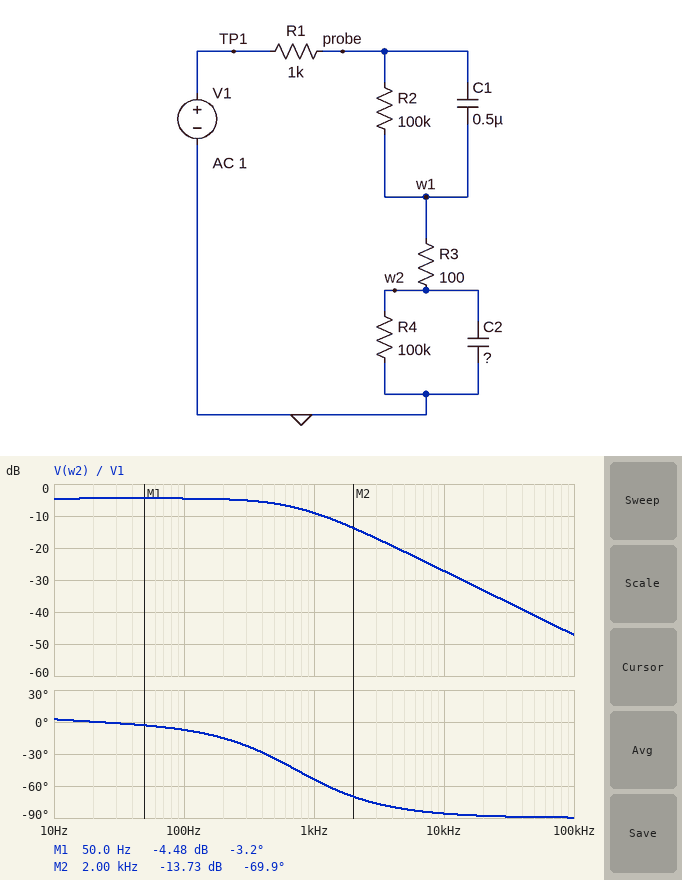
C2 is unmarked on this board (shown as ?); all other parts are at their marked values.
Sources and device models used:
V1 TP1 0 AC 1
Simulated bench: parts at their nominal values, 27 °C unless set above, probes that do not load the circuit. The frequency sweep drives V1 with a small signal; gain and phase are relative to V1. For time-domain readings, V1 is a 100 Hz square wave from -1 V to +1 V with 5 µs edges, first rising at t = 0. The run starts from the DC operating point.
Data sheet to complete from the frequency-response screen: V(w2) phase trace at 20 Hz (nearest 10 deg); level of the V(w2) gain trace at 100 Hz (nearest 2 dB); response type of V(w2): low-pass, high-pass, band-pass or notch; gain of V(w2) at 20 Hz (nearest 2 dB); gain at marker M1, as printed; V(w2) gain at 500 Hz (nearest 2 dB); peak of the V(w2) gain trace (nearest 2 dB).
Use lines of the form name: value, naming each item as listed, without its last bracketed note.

V(w2) phase trace at 20 Hz: 0 deg
level of the V(w2) gain trace at 100 Hz: -4 dB
response type of V(w2): low-pass, high-pass, band-pass or notch: low-pass
gain of V(w2) at 20 Hz: -4 dB
gain at marker M1, as printed: -4.48 dB
V(w2) gain at 500 Hz: -6 dB
peak of the V(w2) gain trace: -4 dB
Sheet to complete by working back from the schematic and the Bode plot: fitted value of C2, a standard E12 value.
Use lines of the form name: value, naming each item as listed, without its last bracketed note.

fitted value of C2, a standard E12 value: 330 nF
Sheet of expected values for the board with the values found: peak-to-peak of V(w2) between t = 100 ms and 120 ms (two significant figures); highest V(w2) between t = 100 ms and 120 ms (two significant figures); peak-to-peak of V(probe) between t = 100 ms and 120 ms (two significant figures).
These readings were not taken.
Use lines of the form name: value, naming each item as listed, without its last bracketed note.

peak-to-peak of V(w2) between t = 100 ms and 120 ms: 1.2 V
highest V(w2) between t = 100 ms and 120 ms: 610 mV
peak-to-peak of V(probe) between t = 100 ms and 120 ms: 2.0 V
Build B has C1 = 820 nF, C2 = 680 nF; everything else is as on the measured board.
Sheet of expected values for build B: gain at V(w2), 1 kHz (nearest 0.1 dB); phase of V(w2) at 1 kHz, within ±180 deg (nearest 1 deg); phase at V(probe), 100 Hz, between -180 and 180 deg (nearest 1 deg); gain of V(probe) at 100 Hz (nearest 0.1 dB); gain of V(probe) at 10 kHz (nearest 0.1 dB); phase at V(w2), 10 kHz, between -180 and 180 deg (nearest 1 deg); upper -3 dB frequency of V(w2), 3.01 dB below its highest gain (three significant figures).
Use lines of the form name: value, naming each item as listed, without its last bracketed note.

gain at V(w2), 1 kHz: -14.1 dB
phase of V(w2) at 1 kHz, within ±180 deg: -69 deg
phase at V(probe), 100 Hz, between -180 and 180 deg: -13 deg
gain of V(probe) at 100 Hz: -0.3 dB
gain of V(probe) at 10 kHz: -20.1 dB
phase at V(w2), 10 kHz, between -180 and 180 deg: -88 deg
upper -3 dB frequency of V(w2), 3.01 dB below its highest gain: 393 Hz
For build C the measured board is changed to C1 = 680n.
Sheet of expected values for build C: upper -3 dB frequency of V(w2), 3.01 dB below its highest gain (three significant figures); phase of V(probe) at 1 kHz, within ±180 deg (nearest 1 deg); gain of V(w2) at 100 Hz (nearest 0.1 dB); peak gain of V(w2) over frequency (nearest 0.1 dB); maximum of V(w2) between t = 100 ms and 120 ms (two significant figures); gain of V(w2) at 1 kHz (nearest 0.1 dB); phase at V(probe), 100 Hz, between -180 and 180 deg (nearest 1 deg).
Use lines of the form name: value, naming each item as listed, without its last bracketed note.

upper -3 dB frequency of V(w2), 3.01 dB below its highest gain: 659 Hz
phase of V(probe) at 1 kHz, within ±180 deg: -49 deg
gain of V(w2) at 100 Hz: -3.6 dB
peak gain of V(w2) over frequency: -3.5 dB
maximum of V(w2) between t = 100 ms and 120 ms: 690 mV
gain of V(w2) at 1 kHz: -8.7 dB
phase at V(probe), 100 Hz, between -180 and 180 deg: -8 deg
